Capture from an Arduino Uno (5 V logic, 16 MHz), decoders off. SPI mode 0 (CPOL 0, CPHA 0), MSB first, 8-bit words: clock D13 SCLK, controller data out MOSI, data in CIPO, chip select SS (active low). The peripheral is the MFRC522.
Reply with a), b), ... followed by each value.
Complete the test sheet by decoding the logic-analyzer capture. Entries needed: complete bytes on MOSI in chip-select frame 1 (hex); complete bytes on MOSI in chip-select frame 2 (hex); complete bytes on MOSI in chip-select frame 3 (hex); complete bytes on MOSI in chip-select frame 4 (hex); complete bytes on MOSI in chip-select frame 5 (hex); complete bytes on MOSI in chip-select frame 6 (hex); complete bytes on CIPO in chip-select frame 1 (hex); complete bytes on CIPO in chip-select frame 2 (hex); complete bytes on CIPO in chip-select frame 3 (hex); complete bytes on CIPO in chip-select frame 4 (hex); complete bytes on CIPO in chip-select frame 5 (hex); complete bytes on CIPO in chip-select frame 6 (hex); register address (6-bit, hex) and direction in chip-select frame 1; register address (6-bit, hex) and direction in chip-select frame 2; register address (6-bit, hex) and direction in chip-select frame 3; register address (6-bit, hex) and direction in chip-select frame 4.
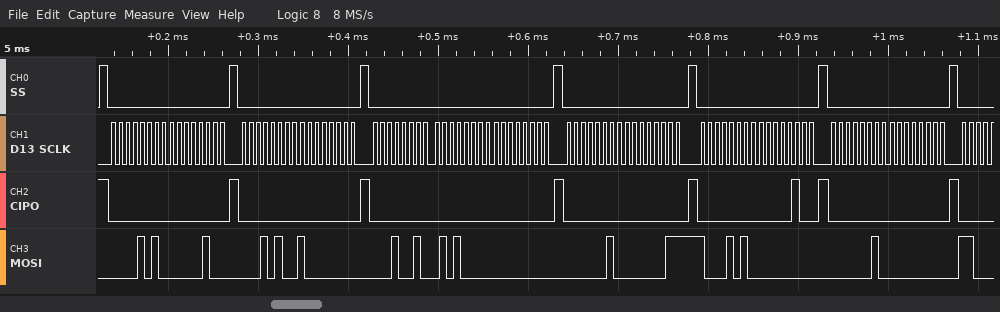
a) 0A 04
b) 14 80
c) 12 50 00
d) 02 03
e) 8A 00
f) 02 00
g) 00 00
h) 00 00
i) 00 00 00
j) 00 00
k) 00 04
l) 00 00
m) 0x05 write
n) 0x0A write
o) 0x09 write
p) 0x01 write
